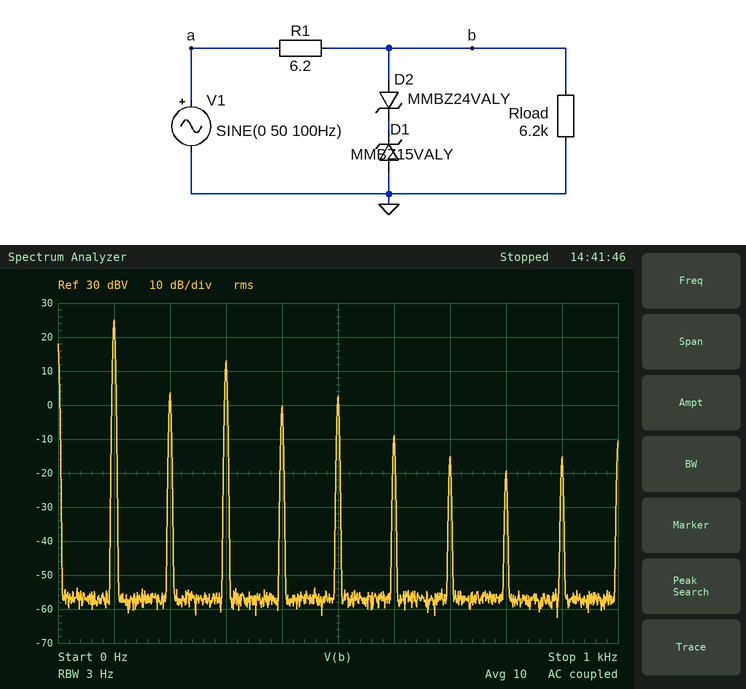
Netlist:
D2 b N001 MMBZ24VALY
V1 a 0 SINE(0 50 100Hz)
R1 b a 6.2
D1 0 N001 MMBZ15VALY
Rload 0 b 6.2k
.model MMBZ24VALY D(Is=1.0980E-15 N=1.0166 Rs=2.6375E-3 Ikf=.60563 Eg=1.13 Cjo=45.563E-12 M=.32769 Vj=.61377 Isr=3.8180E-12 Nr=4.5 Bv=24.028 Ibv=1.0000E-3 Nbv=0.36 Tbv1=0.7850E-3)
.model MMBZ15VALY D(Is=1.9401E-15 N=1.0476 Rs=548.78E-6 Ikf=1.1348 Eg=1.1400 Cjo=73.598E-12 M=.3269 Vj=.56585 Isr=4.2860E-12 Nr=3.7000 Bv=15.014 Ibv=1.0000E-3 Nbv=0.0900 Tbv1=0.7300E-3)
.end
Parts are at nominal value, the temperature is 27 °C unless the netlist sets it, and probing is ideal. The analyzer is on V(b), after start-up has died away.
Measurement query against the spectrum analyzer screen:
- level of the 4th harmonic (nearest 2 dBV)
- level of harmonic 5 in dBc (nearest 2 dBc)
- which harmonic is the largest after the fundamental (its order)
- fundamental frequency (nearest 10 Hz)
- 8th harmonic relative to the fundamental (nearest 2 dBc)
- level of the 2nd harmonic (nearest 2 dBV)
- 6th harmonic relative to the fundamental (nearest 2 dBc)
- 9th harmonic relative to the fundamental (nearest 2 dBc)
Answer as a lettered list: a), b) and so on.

a) 0 dBV
b) -22 dBc
c) 3
d) 100 Hz
e) -44 dBc
f) 4 dBV
g) -34 dBc
h) -40 dBc
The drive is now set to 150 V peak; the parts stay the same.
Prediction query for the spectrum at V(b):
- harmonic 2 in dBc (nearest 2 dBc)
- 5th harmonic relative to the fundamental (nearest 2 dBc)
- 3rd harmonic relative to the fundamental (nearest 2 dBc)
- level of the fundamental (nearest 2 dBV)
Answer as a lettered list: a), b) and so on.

a) -30 dBc
b) -14 dBc
c) -10 dBc
d) 26 dBV
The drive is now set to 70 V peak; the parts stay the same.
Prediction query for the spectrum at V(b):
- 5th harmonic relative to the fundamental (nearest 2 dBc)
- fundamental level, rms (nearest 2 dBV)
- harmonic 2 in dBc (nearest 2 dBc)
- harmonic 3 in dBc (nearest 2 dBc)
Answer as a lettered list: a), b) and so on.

a) -18 dBc
b) 26 dBV
c) -24 dBc
d) -10 dBc
